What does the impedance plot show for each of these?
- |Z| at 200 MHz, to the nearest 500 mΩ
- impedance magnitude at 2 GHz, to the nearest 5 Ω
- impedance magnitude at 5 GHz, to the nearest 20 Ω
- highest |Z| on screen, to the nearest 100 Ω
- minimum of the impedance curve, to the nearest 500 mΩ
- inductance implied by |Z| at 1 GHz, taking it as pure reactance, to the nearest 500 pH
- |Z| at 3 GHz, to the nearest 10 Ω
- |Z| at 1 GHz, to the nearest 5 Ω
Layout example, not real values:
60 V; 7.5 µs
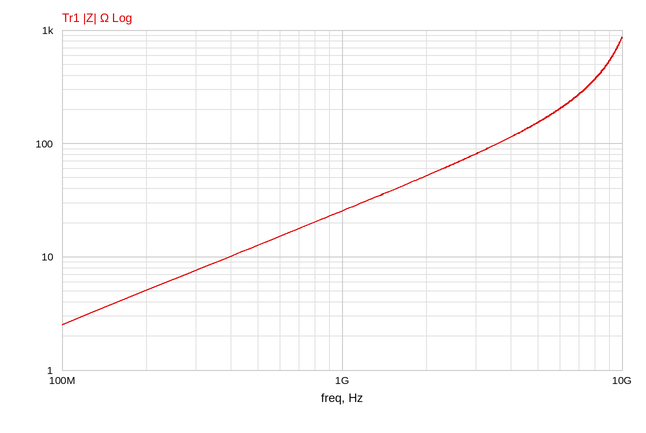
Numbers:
5.0 Ω; 50 Ω; 160 Ω; 900 Ω; 2.5 Ω; 4.0 nH; 80 Ω; 25 Ω
